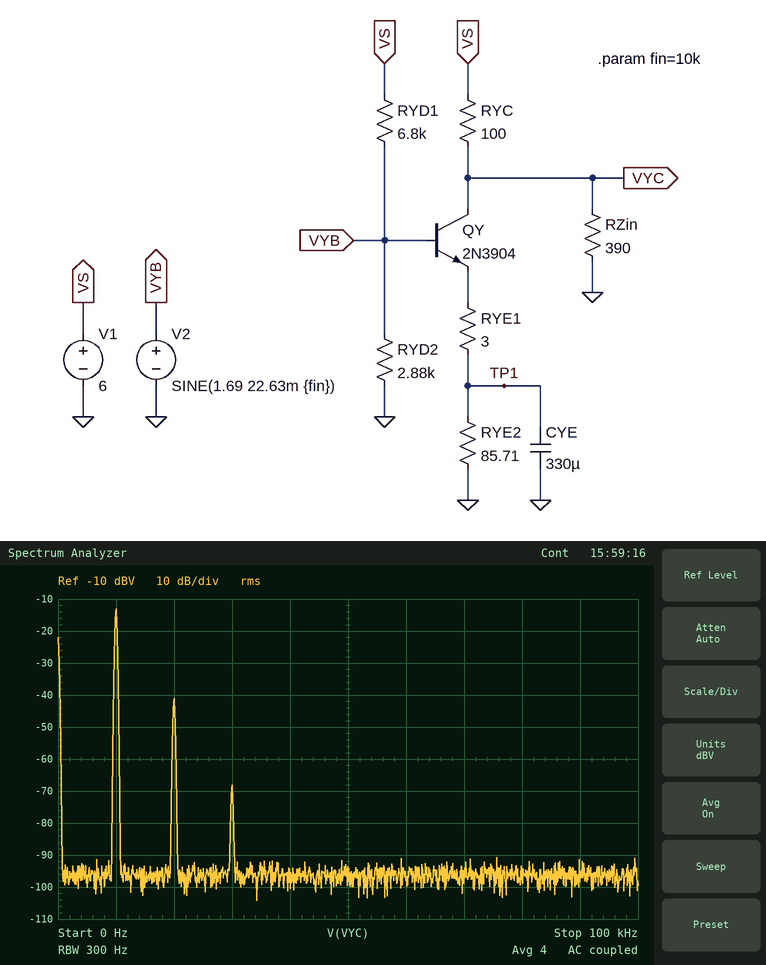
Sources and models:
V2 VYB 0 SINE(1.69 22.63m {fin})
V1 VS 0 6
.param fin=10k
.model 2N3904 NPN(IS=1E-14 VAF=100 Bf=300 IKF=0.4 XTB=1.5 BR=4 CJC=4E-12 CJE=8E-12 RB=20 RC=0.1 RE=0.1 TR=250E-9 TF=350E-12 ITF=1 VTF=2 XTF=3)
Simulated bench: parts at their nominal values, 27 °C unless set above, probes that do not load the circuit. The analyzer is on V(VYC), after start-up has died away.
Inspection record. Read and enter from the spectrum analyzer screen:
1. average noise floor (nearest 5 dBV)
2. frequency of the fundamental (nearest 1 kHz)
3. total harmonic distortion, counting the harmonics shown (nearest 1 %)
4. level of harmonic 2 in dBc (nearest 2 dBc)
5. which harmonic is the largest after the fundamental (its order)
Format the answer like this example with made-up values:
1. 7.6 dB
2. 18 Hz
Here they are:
1. -95 dBV
2. 10 kHz
3. 4 %
4. -28 dBc
5. 2
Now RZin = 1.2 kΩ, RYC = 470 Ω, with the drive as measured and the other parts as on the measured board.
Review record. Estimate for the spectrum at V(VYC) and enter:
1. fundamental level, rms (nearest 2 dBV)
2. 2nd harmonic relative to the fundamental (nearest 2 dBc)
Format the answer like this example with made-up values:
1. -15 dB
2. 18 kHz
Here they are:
1. -38 dBV
2. -10 dBc
